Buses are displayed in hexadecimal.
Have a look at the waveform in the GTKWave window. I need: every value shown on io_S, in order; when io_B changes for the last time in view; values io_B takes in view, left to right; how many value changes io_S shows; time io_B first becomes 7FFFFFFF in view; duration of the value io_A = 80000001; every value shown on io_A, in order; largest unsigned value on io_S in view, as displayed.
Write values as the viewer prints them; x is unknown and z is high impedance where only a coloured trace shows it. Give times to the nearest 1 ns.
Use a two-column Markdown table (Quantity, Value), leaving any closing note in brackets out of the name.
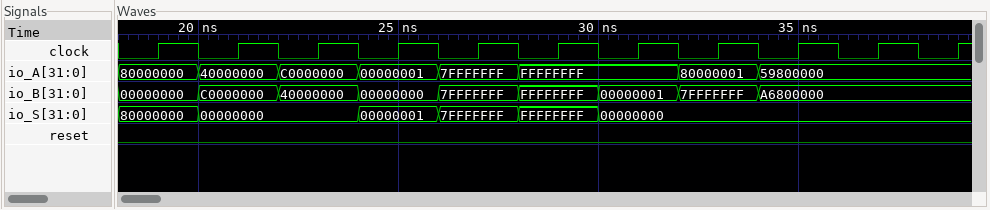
| Quantity | Value |
|---|---|
| every value shown on io_S, in order | 80000000, 00000000, 00000001, 7FFFFFFF, FFFFFFFF, 00000000 |
| when io_B changes for the last time in view | 34 ns |
| values io_B takes in view, left to right | 00000000, C0000000, 40000000, 00000000, 7FFFFFFF, FFFFFFFF, 00000001, 7FFFFFFF, A6800000 |
| how many value changes io_S shows | 5 |
| time io_B first becomes 7FFFFFFF in view | 26 ns |
| duration of the value io_A = 80000001 | 2 ns |
| every value shown on io_A, in order | 80000000, 40000000, C0000000, 00000001, 7FFFFFFF, FFFFFFFF, 80000001, 59800000 |
| largest unsigned value on io_S in view, as displayed | FFFFFFFF |
